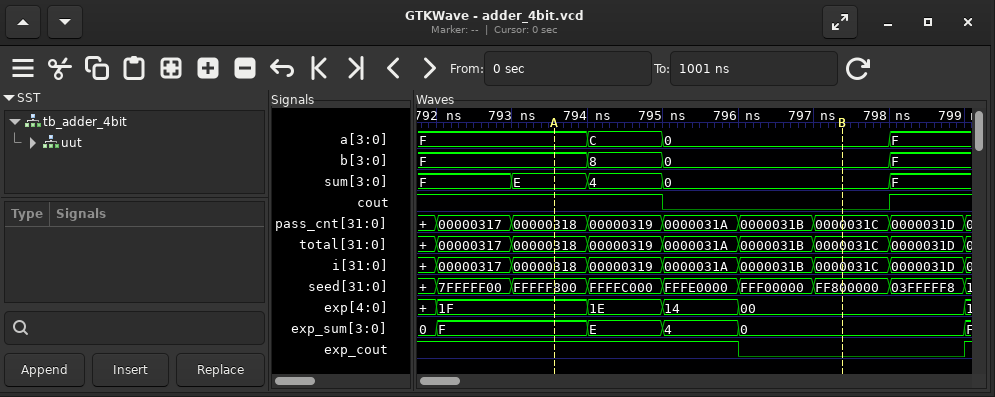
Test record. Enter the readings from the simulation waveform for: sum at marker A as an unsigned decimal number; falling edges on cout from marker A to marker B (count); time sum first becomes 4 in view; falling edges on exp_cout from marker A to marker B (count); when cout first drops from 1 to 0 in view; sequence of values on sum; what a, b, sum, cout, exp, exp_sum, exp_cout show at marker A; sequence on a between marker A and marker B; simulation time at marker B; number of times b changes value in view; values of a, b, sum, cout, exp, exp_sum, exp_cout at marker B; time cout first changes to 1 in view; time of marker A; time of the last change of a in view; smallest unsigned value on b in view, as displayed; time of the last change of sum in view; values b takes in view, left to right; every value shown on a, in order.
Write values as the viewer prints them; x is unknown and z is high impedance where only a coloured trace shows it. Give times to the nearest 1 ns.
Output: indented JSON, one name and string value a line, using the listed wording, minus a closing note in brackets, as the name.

{
  "sum at marker A as an unsigned decimal number": "14",
  "falling edges on cout from marker A to marker B": "1",
  "time sum first becomes 4 in view": "794 ns",
  "falling edges on exp_cout from marker A to marker B": "1",
  "when cout first drops from 1 to 0 in view": "795 ns",
  "sequence of values on sum": "F, E, 4, 0, F",
  "what a, b, sum, cout, exp, exp_sum, exp_cout show at marker A": "a=F, b=F, sum=E, cout=1, exp=1F, exp_sum=F, exp_cout=1",
  "sequence on a between marker A and marker B": "F, C, 0",
  "simulation time at marker B": "797 ns",
  "number of times b changes value in view": "3",
  "values of a, b, sum, cout, exp, exp_sum, exp_cout at marker B": "a=0, b=0, sum=0, cout=0, exp=00, exp_sum=0, exp_cout=0",
  "time cout first changes to 1 in view": "798 ns",
  "time of marker A": "794 ns",
  "time of the last change of a in view": "798 ns",
  "smallest unsigned value on b in view, as displayed": "0",
  "time of the last change of sum in view": "798 ns",
  "values b takes in view, left to right": "F, 8, 0, F",
  "every value shown on a, in order": "F, C, 0, F"
}
